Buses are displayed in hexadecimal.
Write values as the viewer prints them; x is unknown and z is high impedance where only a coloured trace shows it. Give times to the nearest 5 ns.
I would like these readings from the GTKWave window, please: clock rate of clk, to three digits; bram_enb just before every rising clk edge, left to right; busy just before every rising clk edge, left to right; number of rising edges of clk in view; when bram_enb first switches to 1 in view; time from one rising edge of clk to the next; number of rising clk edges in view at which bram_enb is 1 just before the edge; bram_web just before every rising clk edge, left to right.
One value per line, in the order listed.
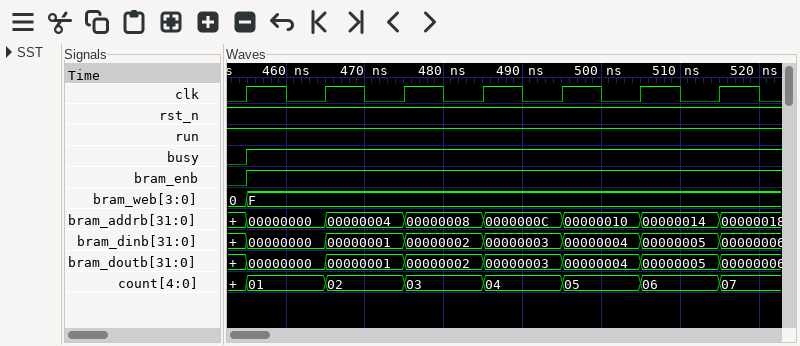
100 MHz
0 1 1 1 1 1 1
0 1 1 1 1 1 1
7
455 ns
10 ns
6
0, F, F, F, F, F, F
